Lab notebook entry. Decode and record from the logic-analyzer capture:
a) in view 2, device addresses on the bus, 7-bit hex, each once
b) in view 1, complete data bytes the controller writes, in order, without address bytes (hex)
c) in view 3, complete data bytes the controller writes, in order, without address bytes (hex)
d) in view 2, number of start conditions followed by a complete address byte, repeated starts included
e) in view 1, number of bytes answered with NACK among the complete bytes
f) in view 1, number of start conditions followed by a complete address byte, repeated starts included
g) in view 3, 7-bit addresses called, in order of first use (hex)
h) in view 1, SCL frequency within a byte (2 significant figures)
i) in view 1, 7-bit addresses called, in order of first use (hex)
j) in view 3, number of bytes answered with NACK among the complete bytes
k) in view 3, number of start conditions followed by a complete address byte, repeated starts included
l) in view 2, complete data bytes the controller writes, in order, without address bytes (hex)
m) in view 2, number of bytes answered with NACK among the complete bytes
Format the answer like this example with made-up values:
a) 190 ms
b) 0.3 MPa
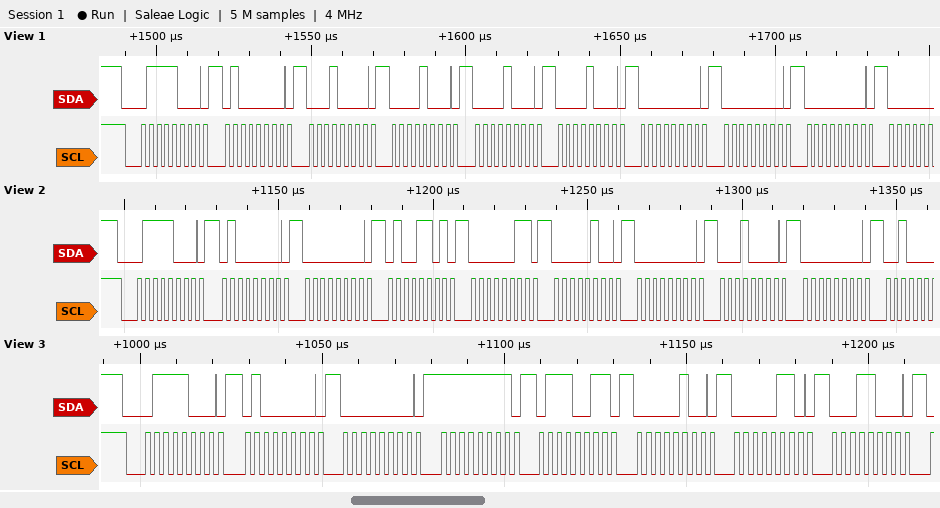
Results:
a) 0x3C
b) 40 10 08 08 08 00 00 00
c) 40 00 FF 73 04 06 18
d) 1
e) 0
f) 1
g) 0x3C
h) 400 kHz
i) 0x3C
j) 0
k) 1
l) 40 00 4D 03 04 00 10 00
m) 0
